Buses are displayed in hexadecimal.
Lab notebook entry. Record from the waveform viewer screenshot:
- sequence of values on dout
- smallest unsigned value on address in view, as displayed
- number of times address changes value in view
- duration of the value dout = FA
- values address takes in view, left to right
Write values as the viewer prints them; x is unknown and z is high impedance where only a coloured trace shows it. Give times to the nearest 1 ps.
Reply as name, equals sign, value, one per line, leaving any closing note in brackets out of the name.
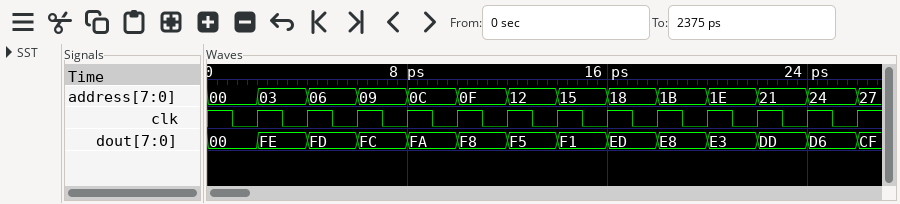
sequence of values on dout = 00, FE, FD, FC, FA, F8, F5, F1, ED, E8, E3, DD, D6, CF
smallest unsigned value on address in view, as displayed = 00
number of times address changes value in view = 13
duration of the value dout = FA = 2 ps
values address takes in view, left to right = 00, 03, 06, 09, 0C, 0F, 12, 15, 18, 1B, 1E, 21, 24, 27
